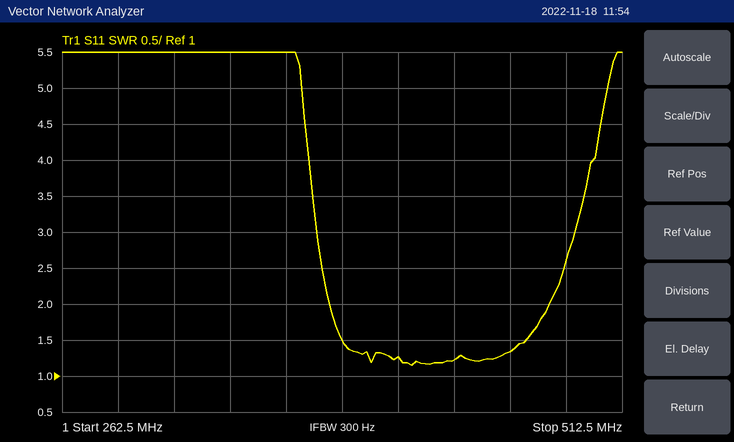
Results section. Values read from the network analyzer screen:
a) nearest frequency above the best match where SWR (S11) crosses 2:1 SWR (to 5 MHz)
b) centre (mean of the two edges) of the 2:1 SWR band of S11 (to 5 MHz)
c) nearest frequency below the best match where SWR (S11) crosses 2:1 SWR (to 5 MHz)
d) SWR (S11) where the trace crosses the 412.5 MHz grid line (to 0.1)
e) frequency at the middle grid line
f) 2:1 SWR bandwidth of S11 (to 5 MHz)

480 MHz
430 MHz
380 MHz
1.3
387.5 MHz
100 MHz
